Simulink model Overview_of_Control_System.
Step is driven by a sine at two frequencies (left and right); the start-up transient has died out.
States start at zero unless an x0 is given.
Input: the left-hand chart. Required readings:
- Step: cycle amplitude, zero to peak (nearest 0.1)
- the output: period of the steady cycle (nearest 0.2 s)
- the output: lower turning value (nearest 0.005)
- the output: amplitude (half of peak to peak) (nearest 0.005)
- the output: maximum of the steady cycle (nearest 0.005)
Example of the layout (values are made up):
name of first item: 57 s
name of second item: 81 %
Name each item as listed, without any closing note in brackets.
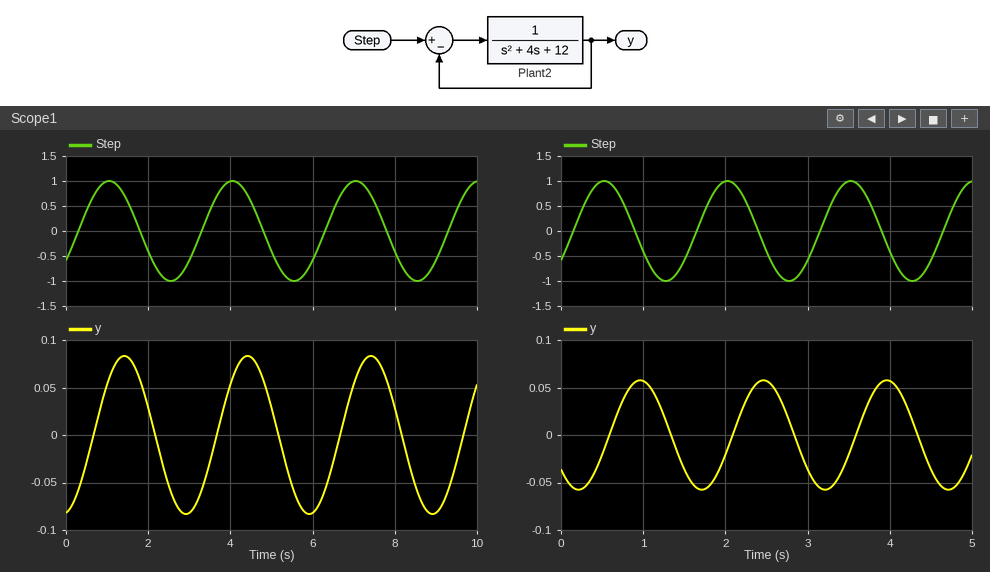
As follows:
Step: cycle amplitude, zero to peak: 1.0
the output: period of the steady cycle: 3.0 s
the output: lower turning value: -0.085
the output: amplitude (half of peak to peak): 0.085
the output: maximum of the steady cycle: 0.085
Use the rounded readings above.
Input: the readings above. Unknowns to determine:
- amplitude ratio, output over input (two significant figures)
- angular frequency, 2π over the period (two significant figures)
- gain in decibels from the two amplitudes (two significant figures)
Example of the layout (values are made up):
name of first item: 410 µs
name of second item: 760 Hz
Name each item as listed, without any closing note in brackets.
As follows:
amplitude ratio, output over input: 0.085
angular frequency, 2π over the period: 2.1 rad/s
gain in decibels from the two amplitudes: -21 dB
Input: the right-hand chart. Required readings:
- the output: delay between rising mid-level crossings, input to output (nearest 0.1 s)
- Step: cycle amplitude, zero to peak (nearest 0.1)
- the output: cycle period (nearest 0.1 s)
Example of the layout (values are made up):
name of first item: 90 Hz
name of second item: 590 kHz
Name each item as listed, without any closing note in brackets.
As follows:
the output: delay between rising mid-level crossings, input to output: 0.4 s
Step: cycle amplitude, zero to peak: 1.0
the output: cycle period: 1.5 s
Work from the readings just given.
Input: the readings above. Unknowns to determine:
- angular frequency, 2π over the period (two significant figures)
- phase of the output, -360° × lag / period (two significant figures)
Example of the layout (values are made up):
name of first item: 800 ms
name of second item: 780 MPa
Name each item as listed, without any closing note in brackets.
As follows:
angular frequency, 2π over the period: 4.2 rad/s
phase of the output, -360° × lag / period: -96°
